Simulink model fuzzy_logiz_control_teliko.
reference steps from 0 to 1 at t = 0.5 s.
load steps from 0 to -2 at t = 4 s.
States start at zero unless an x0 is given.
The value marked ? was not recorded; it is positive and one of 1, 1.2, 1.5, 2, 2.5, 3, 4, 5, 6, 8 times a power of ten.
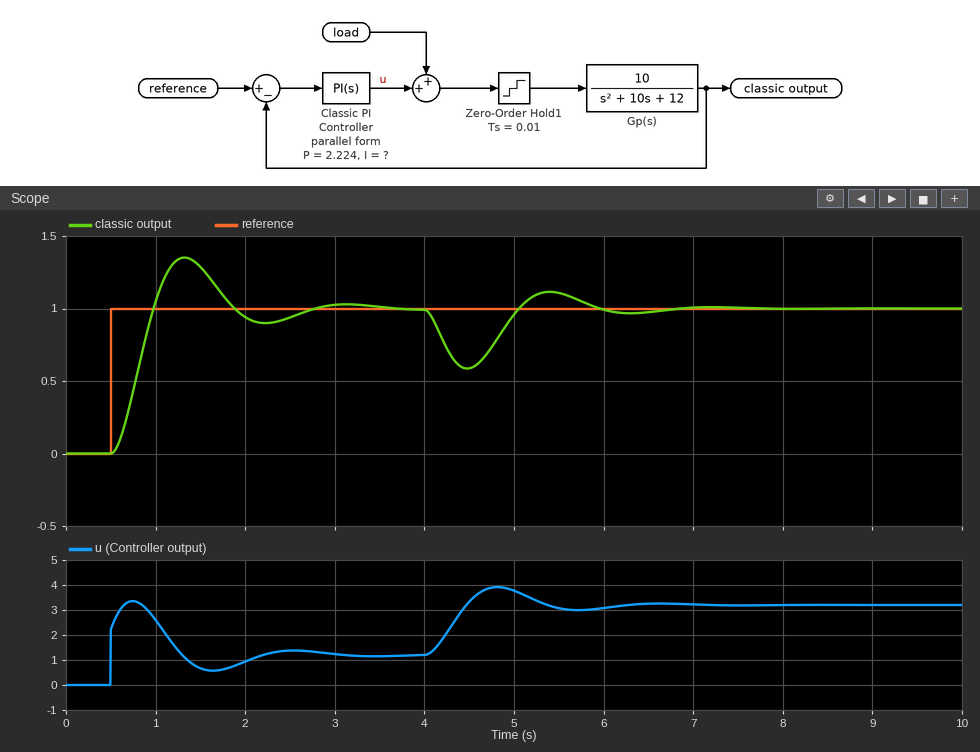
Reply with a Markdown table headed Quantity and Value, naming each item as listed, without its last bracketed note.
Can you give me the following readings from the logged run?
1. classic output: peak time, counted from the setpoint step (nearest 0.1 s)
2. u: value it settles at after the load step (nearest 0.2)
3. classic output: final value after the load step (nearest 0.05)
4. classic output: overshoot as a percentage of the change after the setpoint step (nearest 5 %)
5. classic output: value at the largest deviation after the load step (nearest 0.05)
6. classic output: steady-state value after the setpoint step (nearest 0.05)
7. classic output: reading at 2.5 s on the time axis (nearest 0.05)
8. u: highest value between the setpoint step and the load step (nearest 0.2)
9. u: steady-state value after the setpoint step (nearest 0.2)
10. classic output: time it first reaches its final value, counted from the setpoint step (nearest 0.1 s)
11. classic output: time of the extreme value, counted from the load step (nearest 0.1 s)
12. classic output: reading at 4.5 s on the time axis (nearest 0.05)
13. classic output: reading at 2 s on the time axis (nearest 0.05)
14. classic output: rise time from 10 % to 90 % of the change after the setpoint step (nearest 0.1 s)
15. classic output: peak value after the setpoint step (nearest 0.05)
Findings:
| Quantity | Value |
|---|---|
| classic output: peak time, counted from the setpoint step | 0.8 s |
| u: value it settles at after the load step | 3.2 |
| classic output: final value after the load step | 1.00 |
| classic output: overshoot as a percentage of the change after the setpoint step | 35 % |
| classic output: value at the largest deviation after the load step | 0.60 |
| classic output: steady-state value after the setpoint step | 1.00 |
| classic output: reading at 2.5 s on the time axis | 0.95 |
| u: highest value between the setpoint step and the load step | 3.4 |
| u: steady-state value after the setpoint step | 1.2 |
| classic output: time it first reaches its final value, counted from the setpoint step | 0.5 s |
| classic output: time of the extreme value, counted from the load step | 0.5 s |
| classic output: reading at 4.5 s on the time axis | 0.60 |
| classic output: reading at 2 s on the time axis | 0.95 |
| classic output: rise time from 10 % to 90 % of the change after the setpoint step | 0.3 s |
| classic output: peak value after the setpoint step | 1.35 |
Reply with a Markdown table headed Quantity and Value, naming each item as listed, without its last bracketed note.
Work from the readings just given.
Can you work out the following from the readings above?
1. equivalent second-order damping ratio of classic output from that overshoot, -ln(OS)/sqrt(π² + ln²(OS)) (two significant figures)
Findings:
| Quantity | Value |
|---|---|
| equivalent second-order damping ratio of classic output from that overshoot, -ln(OS)/sqrt(π² + ln²(OS)) | 0.32 |
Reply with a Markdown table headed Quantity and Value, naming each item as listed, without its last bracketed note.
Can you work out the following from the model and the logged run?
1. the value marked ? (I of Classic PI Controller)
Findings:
| Quantity | Value |
|---|---|
| the value marked ? | 10 |
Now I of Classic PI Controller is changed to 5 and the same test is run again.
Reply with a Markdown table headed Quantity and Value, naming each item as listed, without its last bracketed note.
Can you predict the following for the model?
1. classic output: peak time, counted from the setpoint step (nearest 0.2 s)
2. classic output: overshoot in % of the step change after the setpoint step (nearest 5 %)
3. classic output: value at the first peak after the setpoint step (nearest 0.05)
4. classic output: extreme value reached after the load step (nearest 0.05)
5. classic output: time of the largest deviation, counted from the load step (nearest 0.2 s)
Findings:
| Quantity | Value |
|---|---|
| classic output: peak time, counted from the setpoint step | 1.0 s |
| classic output: overshoot in % of the step change after the setpoint step | 10 % |
| classic output: value at the first peak after the setpoint step | 1.10 |
| classic output: extreme value reached after the load step | 0.55 |
| classic output: time of the largest deviation, counted from the load step | 0.6 s |
